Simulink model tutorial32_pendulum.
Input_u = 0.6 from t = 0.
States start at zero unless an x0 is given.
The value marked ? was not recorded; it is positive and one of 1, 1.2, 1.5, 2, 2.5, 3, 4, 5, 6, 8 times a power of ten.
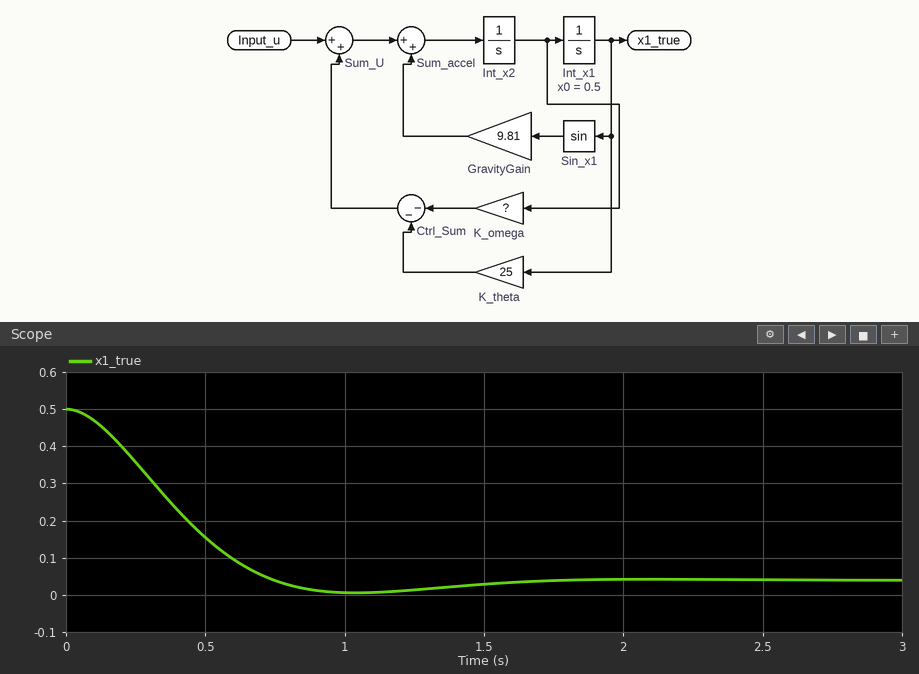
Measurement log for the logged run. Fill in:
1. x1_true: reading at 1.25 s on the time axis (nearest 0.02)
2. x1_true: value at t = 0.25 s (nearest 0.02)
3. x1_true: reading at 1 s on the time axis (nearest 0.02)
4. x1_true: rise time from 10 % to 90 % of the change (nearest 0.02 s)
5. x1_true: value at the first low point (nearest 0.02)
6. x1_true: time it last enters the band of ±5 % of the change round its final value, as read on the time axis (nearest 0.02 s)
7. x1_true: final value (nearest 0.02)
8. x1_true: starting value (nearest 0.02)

0.02
0.36
0.00
0.50 s
0.00
1.30 s
0.04
0.50
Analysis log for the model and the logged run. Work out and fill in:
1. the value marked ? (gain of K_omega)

5
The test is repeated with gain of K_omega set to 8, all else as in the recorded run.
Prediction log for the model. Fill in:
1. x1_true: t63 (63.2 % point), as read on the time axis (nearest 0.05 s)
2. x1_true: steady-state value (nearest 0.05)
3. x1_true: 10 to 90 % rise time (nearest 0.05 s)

0.55 s
0.05
0.90 s
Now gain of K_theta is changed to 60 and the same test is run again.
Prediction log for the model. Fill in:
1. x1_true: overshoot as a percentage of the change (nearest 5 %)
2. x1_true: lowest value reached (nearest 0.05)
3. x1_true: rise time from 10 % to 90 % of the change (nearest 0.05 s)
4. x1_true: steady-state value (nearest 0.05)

30 %
-0.15
0.20 s
0.00
